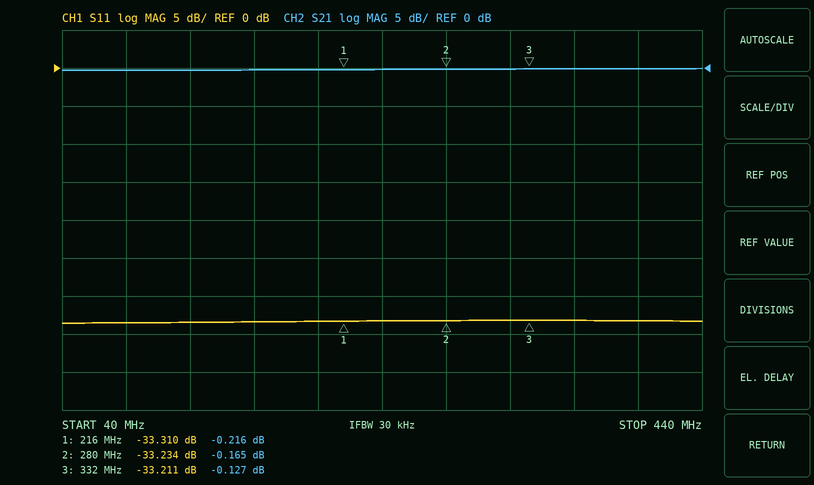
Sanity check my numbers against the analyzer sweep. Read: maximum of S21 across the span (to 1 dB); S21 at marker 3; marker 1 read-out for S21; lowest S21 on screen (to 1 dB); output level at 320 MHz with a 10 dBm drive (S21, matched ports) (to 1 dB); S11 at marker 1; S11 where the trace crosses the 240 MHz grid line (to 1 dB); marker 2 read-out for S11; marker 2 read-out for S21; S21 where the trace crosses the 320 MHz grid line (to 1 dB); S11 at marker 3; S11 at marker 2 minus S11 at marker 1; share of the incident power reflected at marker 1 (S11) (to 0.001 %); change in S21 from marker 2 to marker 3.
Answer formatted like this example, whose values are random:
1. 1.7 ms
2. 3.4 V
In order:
1. 0 dB
2. -0.127 dB
3. -0.216 dB
4. 0 dB
5. 10 dBm
6. -33.310 dB
7. -33 dB
8. -33.234 dB
9. -0.165 dB
10. 0 dB
11. -33.211 dB
12. 0.076 dB
13. 0.047 %
14. 0.038 dB
